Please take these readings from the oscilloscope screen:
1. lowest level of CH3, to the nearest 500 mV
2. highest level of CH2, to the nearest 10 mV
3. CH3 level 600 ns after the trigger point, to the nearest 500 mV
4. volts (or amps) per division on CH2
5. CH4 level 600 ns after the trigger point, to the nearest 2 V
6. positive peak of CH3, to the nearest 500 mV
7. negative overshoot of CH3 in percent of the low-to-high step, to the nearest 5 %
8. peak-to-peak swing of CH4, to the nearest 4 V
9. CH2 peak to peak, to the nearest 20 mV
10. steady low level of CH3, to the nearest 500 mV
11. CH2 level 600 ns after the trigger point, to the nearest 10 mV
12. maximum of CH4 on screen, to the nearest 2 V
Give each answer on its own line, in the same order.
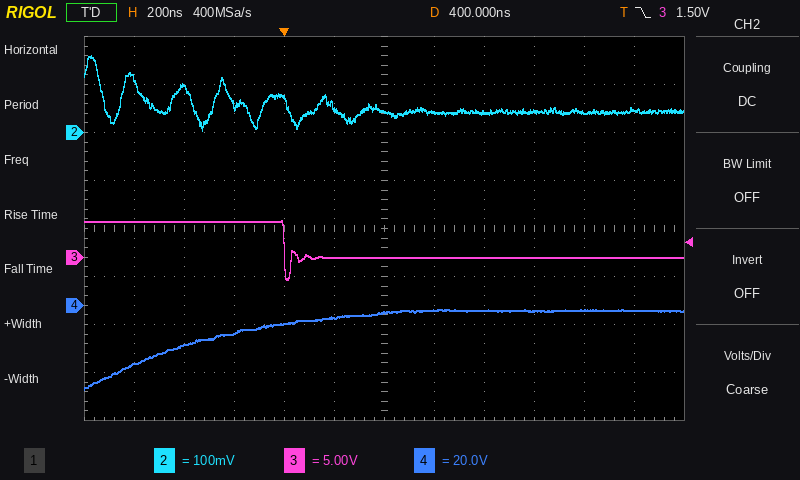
-2.5 V
160 mV
0.0 V
100 mV
-2 V
4.0 V
60 %
32 V
160 mV
0.0 V
40 mV
-2 V
